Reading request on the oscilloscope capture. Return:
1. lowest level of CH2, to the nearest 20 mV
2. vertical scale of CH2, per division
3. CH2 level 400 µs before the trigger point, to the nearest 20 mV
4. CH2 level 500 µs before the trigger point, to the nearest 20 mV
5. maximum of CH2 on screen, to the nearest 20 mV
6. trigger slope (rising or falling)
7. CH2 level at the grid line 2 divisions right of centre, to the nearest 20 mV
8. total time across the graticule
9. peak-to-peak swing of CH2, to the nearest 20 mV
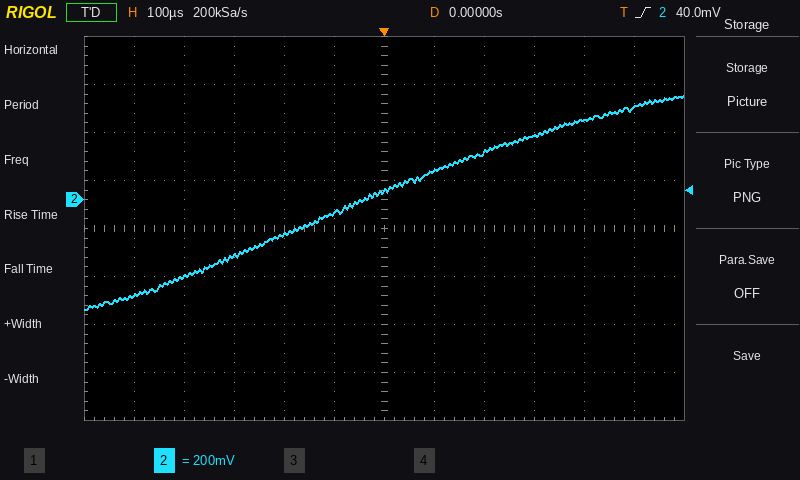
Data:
-460 mV
200 mV
-320 mV
-400 mV
440 mV
rising
200 mV
1.2 ms
900 mV
